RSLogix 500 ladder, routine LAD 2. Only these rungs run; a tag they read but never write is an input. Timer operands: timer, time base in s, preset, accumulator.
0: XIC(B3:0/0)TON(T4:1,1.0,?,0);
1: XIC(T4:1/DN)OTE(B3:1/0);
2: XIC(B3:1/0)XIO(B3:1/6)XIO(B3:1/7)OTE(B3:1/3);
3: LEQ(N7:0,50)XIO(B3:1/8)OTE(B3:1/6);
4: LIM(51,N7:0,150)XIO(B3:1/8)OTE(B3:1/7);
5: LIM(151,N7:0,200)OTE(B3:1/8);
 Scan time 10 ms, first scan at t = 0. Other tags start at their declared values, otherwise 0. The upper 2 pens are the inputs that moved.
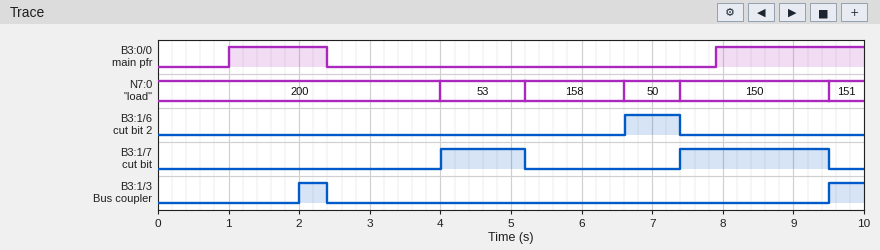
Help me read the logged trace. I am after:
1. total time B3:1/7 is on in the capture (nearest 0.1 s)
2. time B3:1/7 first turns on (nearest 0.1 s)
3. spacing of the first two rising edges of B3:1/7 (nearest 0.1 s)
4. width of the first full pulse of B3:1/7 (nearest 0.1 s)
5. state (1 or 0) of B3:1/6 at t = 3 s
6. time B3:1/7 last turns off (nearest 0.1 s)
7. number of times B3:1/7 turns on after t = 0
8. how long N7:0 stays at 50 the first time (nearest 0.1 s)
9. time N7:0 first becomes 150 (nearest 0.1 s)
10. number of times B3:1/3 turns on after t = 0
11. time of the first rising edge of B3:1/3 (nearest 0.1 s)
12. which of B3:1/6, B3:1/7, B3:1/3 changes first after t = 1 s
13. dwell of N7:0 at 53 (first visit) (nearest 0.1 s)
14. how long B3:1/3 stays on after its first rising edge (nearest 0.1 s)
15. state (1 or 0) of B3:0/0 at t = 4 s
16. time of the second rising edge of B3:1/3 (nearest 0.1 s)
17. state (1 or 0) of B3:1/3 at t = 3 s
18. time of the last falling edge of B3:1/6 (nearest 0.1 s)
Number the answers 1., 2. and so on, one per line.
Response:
1. 3.3 s
2. 4.0 s
3. 3.4 s
4. 1.2 s
5. 0
6. 9.5 s
7. 2
8. 0.8 s
9. 7.4 s
10. 2
11. 2.0 s
12. B3:1/3
13. 1.2 s
14. 0.4 s
15. 0
16. 9.5 s
17. 0
18. 7.4 s
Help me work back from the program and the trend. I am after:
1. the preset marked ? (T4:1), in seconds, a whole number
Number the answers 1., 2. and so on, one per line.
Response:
1. 1 s
